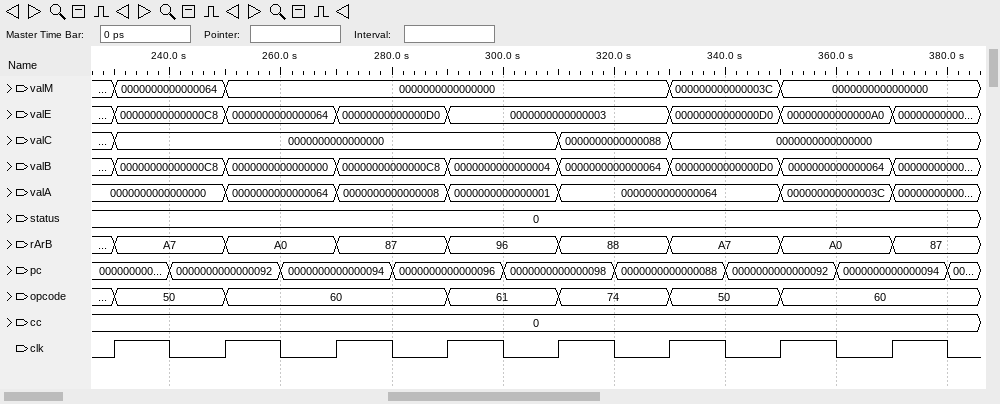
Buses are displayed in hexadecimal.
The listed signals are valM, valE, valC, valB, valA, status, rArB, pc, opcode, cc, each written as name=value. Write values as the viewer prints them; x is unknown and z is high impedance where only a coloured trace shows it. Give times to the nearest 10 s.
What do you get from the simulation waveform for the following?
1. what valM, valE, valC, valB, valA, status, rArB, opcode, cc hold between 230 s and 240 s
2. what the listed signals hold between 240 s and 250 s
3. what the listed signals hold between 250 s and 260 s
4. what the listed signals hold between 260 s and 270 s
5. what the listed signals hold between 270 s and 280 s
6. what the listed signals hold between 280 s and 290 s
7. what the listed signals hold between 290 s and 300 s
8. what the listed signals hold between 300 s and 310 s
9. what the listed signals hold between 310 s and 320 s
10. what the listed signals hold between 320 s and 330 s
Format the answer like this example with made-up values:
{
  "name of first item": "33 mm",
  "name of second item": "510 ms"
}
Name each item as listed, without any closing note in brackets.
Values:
{
  "what valM, valE, valC, valB, valA, status, rArB, opcode, cc hold between 230 s and 240 s": "valM=0000000000000064, valE=00000000000000C8, valC=0000000000000000, valB=00000000000000C8, valA=0000000000000000, status=0, rArB=A7, opcode=50, cc=0",
  "what the listed signals hold between 240 s and 250 s": "valM=0000000000000064, valE=00000000000000C8, valC=0000000000000000, valB=00000000000000C8, valA=0000000000000000, status=0, rArB=A7, pc=0000000000000092, opcode=50, cc=0",
  "what the listed signals hold between 250 s and 260 s": "valM=0000000000000000, valE=0000000000000064, valC=0000000000000000, valB=0000000000000000, valA=0000000000000064, status=0, rArB=A0, pc=0000000000000092, opcode=60, cc=0",
  "what the listed signals hold between 260 s and 270 s": "valM=0000000000000000, valE=0000000000000064, valC=0000000000000000, valB=0000000000000000, valA=0000000000000064, status=0, rArB=A0, pc=0000000000000094, opcode=60, cc=0",
  "what the listed signals hold between 270 s and 280 s": "valM=0000000000000000, valE=00000000000000D0, valC=0000000000000000, valB=00000000000000C8, valA=0000000000000008, status=0, rArB=87, pc=0000000000000094, opcode=60, cc=0",
  "what the listed signals hold between 280 s and 290 s": "valM=0000000000000000, valE=00000000000000D0, valC=0000000000000000, valB=00000000000000C8, valA=0000000000000008, status=0, rArB=87, pc=0000000000000096, opcode=60, cc=0",
  "what the listed signals hold between 290 s and 300 s": "valM=0000000000000000, valE=0000000000000003, valC=0000000000000000, valB=0000000000000004, valA=0000000000000001, status=0, rArB=96, pc=0000000000000096, opcode=61, cc=0",
  "what the listed signals hold between 300 s and 310 s": "valM=0000000000000000, valE=0000000000000003, valC=0000000000000000, valB=0000000000000004, valA=0000000000000001, status=0, rArB=96, pc=0000000000000098, opcode=61, cc=0",
  "what the listed signals hold between 310 s and 320 s": "valM=0000000000000000, valE=0000000000000003, valC=0000000000000088, valB=0000000000000064, valA=0000000000000064, status=0, rArB=88, pc=0000000000000098, opcode=74, cc=0",
  "what the listed signals hold between 320 s and 330 s": "valM=0000000000000000, valE=0000000000000003, valC=0000000000000088, valB=0000000000000064, valA=0000000000000064, status=0, rArB=88, pc=0000000000000088, opcode=74, cc=0"
}
